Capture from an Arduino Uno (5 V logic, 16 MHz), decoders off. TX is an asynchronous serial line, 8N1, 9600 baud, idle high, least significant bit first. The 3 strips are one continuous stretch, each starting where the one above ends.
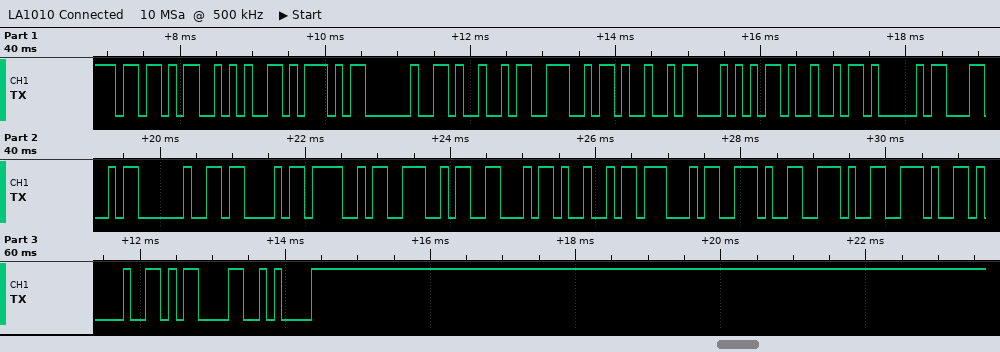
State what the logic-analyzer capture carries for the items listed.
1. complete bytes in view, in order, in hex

0x5B 0x2A 0x5D 0x20 0x49 0x4E 0x49 0x54 0x49 0x41 0x4C 0x20 0x43 0x4F 0x4E 0x46 0x49 0x47 0x2E 0x2E 0x2E 0x21 0x0D 0x0A
